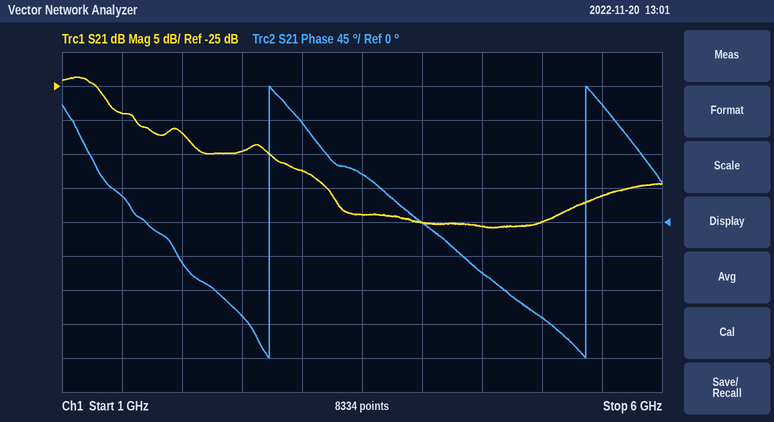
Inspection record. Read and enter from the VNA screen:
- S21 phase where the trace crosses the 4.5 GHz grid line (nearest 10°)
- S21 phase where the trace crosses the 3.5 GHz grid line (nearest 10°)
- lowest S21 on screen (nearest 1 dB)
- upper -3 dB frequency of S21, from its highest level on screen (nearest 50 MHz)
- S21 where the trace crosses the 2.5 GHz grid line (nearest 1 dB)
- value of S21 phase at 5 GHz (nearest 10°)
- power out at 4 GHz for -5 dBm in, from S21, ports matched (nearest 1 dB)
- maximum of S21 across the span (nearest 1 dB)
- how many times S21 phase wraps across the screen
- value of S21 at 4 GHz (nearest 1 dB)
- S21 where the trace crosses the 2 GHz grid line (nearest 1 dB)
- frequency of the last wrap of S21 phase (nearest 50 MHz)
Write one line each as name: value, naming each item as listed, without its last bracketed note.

S21 phase where the trace crosses the 4.5 GHz grid line: -70°
S21 phase where the trace crosses the 3.5 GHz grid line: 60°
lowest S21 on screen: -46 dB
upper -3 dB frequency of S21, from its highest level on screen: 1.35 GHz
S21 where the trace crosses the 2.5 GHz grid line: -35 dB
value of S21 phase at 5 GHz: -130°
power out at 4 GHz for -5 dBm in, from S21, ports matched: -50 dBm
maximum of S21 across the span: -24 dB
how many times S21 phase wraps across the screen: 2
value of S21 at 4 GHz: -45 dB
S21 where the trace crosses the 2 GHz grid line: -32 dB
frequency of the last wrap of S21 phase: 5.35 GHz
